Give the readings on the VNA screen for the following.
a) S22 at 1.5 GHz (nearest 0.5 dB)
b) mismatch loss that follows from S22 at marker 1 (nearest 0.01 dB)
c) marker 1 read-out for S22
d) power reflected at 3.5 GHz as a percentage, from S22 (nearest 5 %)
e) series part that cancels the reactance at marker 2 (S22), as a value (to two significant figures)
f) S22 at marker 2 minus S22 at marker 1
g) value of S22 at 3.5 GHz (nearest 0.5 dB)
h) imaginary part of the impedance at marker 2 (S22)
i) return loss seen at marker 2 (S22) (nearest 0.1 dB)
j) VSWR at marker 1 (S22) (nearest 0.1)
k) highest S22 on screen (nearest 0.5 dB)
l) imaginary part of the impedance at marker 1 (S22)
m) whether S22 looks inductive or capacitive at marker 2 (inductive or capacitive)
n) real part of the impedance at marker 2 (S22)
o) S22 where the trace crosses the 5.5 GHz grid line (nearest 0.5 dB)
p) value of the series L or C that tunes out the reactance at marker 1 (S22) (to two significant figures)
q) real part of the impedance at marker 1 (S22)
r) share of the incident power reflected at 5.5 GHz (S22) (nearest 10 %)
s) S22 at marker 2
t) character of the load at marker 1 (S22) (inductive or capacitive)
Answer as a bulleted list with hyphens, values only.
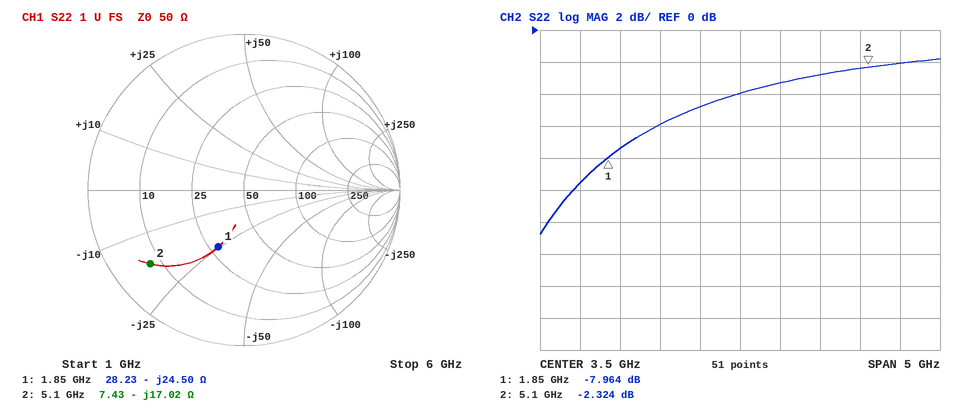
- -9.5 dB
- 0.76 dB
- -7.964 dB
- 40 %
- 530 pH
- 5.640 dB
- -4.0 dB
- -17.02 Ω
- 2.3 dB
- 2.3
- -2.0 dB
- -24.50 Ω
- capacitive
- 7.43 Ω
- -2.0 dB
- 2.1 nH
- 28.23 Ω
- 60 %
- -2.324 dB
- capacitive
